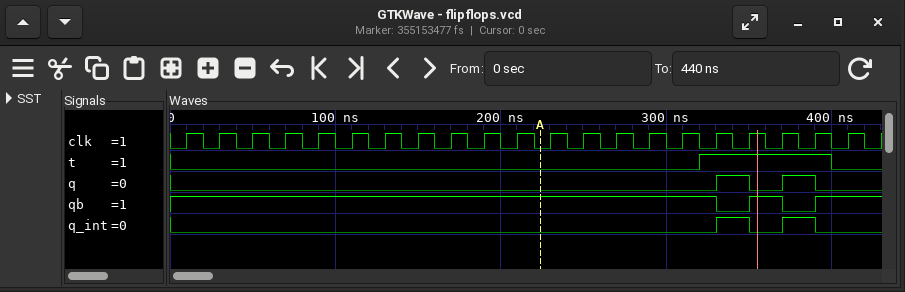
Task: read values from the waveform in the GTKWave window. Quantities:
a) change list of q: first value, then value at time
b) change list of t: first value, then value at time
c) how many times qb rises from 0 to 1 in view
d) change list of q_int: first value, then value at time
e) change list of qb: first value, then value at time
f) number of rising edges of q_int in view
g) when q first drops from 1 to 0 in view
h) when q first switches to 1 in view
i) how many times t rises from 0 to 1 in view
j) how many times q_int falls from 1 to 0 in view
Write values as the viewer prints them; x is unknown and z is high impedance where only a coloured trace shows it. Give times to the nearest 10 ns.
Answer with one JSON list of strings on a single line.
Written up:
["0, 1 at 330 ns, 0 at 350 ns, 1 at 370 ns, 0 at 390 ns", "0, 1 at 320 ns, 0 at 400 ns", "2", "0, 1 at 330 ns, 0 at 350 ns, 1 at 370 ns, 0 at 390 ns", "1, 0 at 330 ns, 1 at 350 ns, 0 at 370 ns, 1 at 390 ns", "2", "350 ns", "330 ns", "1", "2"]
